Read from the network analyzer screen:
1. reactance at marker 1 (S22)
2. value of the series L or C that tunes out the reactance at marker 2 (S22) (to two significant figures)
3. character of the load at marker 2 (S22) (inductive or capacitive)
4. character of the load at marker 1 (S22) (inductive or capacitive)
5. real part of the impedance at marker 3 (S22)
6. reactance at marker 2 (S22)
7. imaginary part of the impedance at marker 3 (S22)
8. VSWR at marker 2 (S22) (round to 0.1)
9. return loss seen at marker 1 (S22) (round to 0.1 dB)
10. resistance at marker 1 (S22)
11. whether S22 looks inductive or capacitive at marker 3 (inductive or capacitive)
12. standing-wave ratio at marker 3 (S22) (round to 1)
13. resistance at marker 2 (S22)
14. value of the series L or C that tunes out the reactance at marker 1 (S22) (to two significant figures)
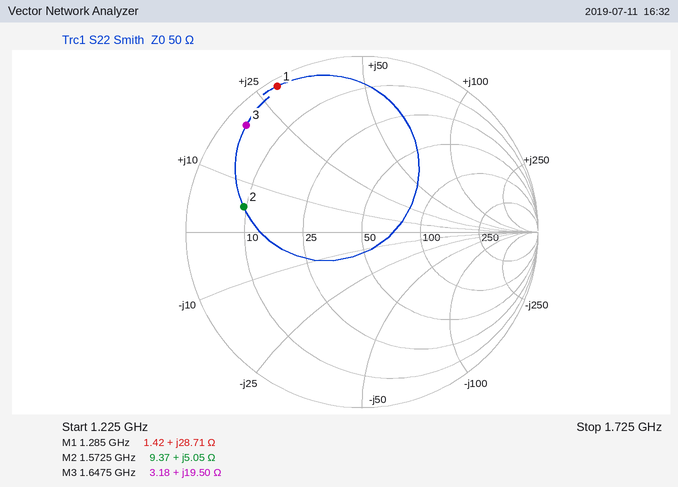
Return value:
+28.71 Ω
20 pF
inductive
inductive
3.18 Ω
+5.05 Ω
+19.50 Ω
5.4
0.4 dB
1.42 Ω
inductive
18
9.37 Ω
4.3 pF
